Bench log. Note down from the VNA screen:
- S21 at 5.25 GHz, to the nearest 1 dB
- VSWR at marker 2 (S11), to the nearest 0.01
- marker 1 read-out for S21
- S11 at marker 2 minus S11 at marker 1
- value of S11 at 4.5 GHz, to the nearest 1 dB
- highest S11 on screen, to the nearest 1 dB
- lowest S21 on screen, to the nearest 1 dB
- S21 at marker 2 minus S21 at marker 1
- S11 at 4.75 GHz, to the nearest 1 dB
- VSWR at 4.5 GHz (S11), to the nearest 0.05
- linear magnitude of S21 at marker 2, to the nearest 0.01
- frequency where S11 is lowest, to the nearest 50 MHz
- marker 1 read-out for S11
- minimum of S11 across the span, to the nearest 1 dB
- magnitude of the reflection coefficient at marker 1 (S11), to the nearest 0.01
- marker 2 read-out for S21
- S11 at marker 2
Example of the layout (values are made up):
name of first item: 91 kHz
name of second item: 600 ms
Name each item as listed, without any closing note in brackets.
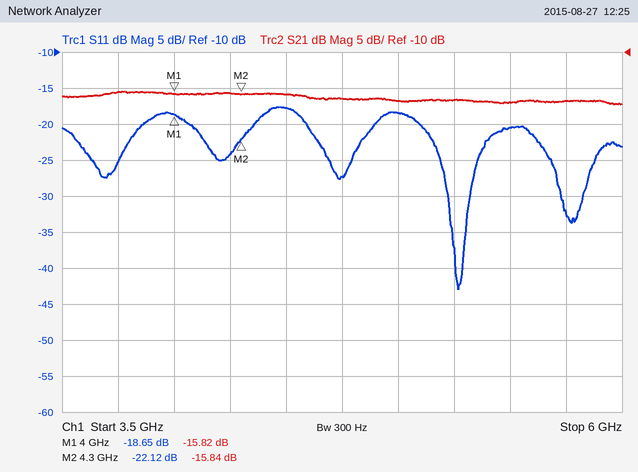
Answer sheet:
S21 at 5.25 GHz, to the nearest 1 dB: -17 dB
VSWR at marker 2 (S11), to the nearest 0.01: 1.17
marker 1 read-out for S21: -15.82 dB
S11 at marker 2 minus S11 at marker 1: -3.47 dB
value of S11 at 4.5 GHz, to the nearest 1 dB: -18 dB
highest S11 on screen, to the nearest 1 dB: -18 dB
lowest S21 on screen, to the nearest 1 dB: -17 dB
S21 at marker 2 minus S21 at marker 1: -0.02 dB
S11 at 4.75 GHz, to the nearest 1 dB: -27 dB
VSWR at 4.5 GHz (S11), to the nearest 0.05: 1.30
linear magnitude of S21 at marker 2, to the nearest 0.01: 0.16
frequency where S11 is lowest, to the nearest 50 MHz: 5.25 GHz
marker 1 read-out for S11: -18.65 dB
minimum of S11 across the span, to the nearest 1 dB: -43 dB
magnitude of the reflection coefficient at marker 1 (S11), to the nearest 0.01: 0.12
marker 2 read-out for S21: -15.84 dB
S11 at marker 2: -22.12 dB
